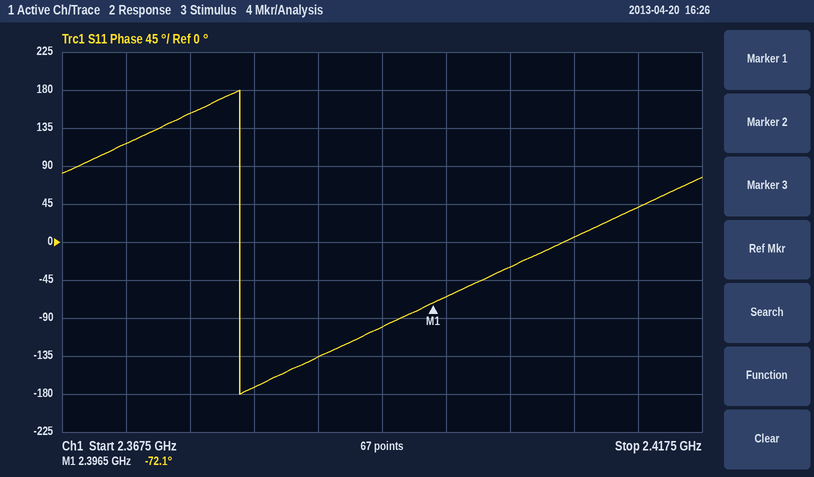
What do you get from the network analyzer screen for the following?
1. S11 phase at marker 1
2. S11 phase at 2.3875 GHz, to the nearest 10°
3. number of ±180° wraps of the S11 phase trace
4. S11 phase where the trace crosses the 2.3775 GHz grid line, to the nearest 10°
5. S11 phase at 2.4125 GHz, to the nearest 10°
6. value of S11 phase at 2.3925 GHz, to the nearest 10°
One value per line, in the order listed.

-72.1°
-140°
1
150°
40°
-100°
